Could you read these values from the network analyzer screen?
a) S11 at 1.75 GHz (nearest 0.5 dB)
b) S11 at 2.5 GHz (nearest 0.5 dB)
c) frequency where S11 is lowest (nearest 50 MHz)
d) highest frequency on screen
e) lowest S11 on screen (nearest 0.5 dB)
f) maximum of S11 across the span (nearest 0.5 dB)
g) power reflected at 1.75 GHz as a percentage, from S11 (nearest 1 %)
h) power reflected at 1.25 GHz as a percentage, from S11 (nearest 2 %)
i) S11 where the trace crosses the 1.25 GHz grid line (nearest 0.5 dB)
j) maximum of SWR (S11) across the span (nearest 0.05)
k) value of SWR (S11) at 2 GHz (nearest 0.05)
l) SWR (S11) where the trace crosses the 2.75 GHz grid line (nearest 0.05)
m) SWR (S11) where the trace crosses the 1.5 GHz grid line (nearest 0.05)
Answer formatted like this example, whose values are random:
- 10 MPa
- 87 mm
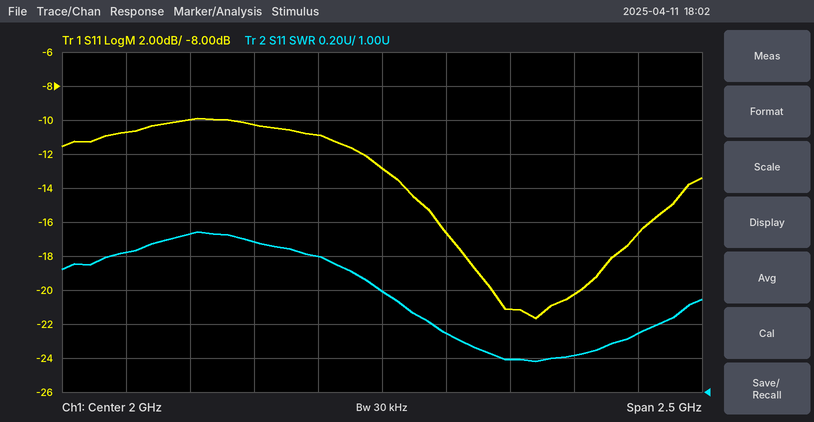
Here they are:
- -11.0 dB
- -21.0 dB
- 2.60 GHz
- 3.25 GHz
- -21.5 dB
- -10.0 dB
- 8 %
- 10 %
- -10.0 dB
- 1.95
- 1.60
- 1.20
- 1.90
